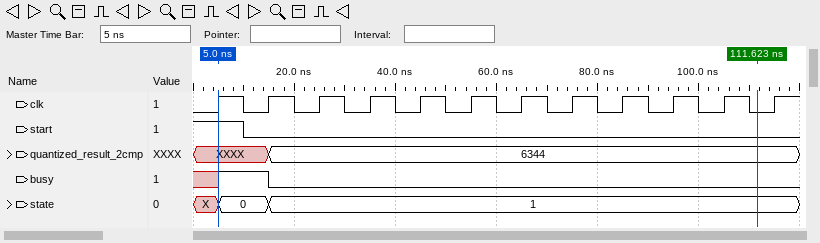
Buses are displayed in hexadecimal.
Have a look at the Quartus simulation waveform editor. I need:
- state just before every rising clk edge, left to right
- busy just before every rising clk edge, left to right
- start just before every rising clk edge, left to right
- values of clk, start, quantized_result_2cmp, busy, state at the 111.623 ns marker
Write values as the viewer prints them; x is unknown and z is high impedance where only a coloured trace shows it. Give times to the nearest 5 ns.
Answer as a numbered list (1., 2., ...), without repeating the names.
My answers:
1. X, 0, 1, 1, 1, 1, 1, 1, 1, 1, 1, 1
2. x 1 0 0 0 0 0 0 0 0 0 0
3. 1 0 0 0 0 0 0 0 0 0 0 0
4. clk=0, start=0, quantized_result_2cmp=6344, busy=0, state=1
